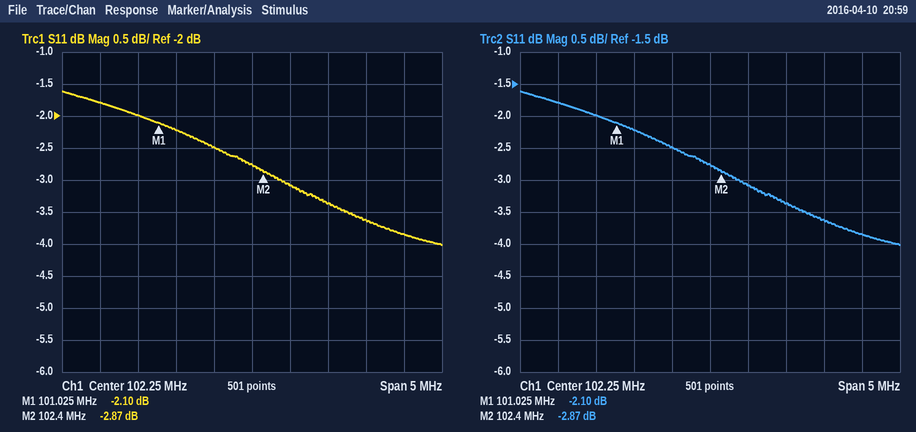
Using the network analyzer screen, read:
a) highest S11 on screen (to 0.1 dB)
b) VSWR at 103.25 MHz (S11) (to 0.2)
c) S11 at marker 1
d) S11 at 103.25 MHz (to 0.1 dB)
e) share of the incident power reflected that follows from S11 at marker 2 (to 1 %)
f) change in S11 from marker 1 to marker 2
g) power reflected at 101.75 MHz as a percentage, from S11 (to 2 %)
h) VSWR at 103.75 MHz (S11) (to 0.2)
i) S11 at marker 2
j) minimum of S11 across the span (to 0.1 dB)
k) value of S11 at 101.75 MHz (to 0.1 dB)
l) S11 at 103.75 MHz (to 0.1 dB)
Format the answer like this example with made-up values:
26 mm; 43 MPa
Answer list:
-1.6 dB; 5.2; -2.10 dB; -3.4 dB; 52 %; -0.77 dB; 56 %; 4.8; -2.87 dB; -4.0 dB; -2.5 dB; -3.6 dB
